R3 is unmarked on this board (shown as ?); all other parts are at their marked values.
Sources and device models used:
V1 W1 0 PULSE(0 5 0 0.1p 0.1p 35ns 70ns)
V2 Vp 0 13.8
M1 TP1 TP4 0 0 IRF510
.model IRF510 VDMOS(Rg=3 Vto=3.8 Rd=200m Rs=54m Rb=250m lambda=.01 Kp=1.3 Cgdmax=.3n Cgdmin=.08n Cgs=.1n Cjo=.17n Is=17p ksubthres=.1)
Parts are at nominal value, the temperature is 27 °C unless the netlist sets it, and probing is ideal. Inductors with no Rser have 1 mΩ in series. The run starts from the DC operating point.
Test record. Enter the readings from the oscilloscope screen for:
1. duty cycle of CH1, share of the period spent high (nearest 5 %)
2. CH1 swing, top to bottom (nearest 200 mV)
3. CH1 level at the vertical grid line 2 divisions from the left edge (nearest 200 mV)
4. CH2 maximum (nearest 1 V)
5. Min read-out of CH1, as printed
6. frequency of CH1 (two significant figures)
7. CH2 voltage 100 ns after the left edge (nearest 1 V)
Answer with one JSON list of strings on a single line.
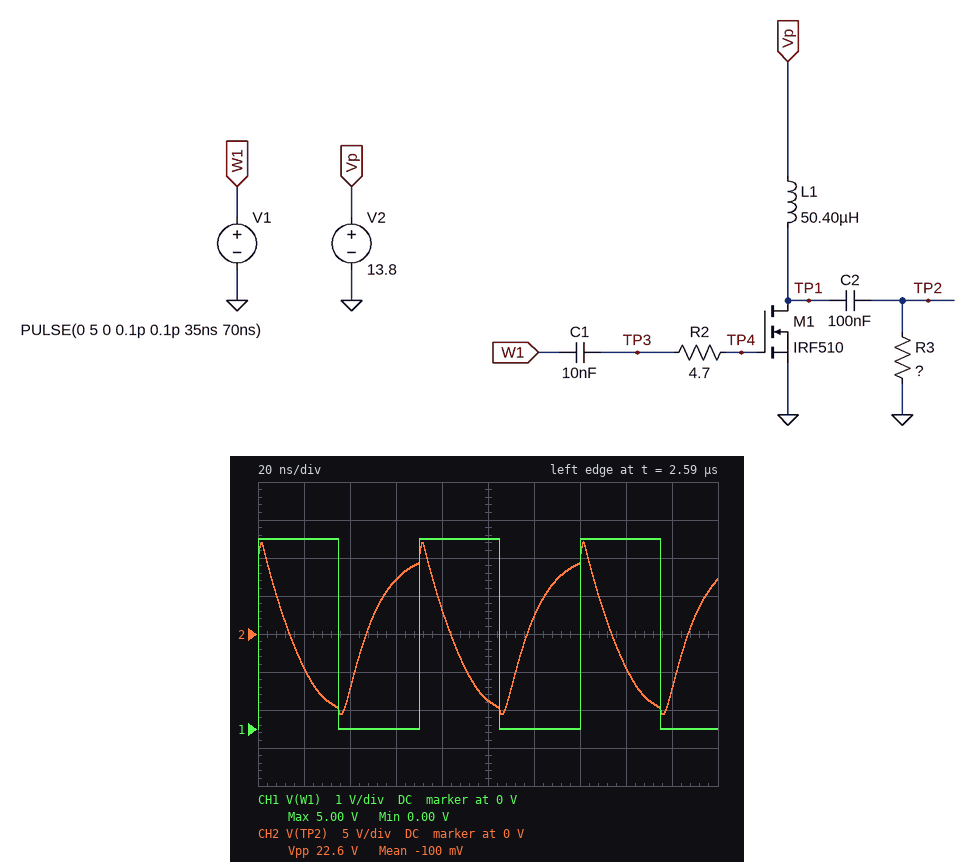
["50 %", "5.0 V", "0 V", "12 V", "0.00 V", "14 MHz", "-9 V"]
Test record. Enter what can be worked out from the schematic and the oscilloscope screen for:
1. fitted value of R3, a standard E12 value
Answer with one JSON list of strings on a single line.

["100 Ω"]
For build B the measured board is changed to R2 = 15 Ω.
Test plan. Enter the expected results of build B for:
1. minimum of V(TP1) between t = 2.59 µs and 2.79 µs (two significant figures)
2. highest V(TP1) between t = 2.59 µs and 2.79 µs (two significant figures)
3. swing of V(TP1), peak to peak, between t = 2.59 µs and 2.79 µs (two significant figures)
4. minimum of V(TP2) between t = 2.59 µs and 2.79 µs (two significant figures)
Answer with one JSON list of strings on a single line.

["6.1 V", "21 V", "15 V", "-3.6 V"]
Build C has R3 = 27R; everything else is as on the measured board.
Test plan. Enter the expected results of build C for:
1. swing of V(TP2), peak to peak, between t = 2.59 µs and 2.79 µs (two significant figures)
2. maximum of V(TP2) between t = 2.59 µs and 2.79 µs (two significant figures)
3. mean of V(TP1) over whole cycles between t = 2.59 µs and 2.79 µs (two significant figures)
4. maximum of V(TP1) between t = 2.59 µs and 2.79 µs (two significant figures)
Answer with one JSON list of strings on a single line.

["14 V", "6.3 V", "12 V", "18 V"]
